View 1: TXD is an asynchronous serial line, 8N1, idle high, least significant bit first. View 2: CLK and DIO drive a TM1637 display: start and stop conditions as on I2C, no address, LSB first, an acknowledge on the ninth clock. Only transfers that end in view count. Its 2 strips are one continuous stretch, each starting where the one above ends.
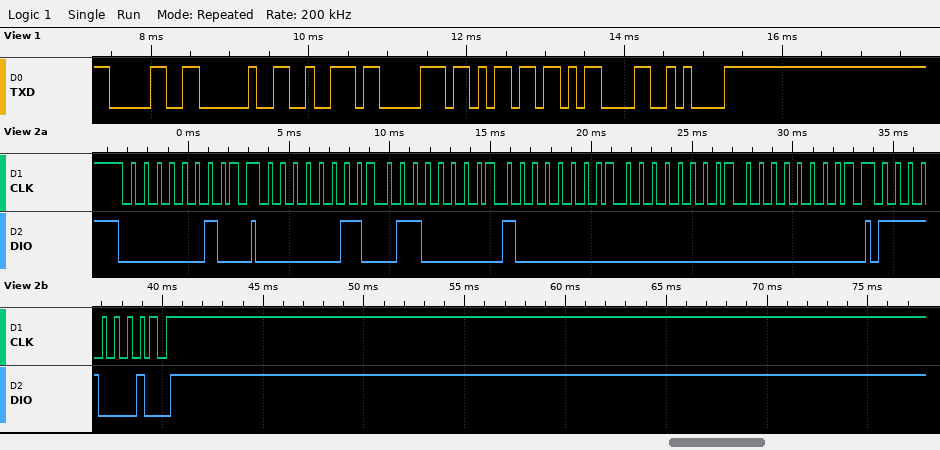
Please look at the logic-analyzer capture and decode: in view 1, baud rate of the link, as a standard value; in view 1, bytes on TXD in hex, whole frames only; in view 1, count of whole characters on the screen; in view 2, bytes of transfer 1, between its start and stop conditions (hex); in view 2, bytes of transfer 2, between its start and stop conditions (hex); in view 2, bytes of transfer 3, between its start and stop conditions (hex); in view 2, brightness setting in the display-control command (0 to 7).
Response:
9600 baud
30 20 72 70 6D 0D 0A
7
40
C0 06 01 00 00
8F
7
